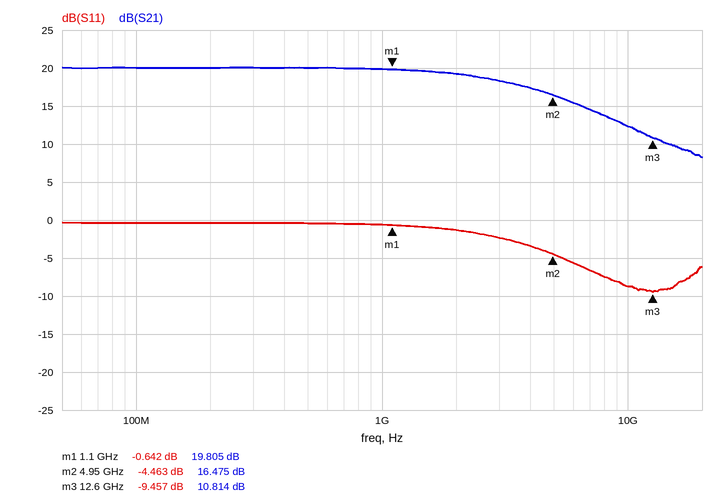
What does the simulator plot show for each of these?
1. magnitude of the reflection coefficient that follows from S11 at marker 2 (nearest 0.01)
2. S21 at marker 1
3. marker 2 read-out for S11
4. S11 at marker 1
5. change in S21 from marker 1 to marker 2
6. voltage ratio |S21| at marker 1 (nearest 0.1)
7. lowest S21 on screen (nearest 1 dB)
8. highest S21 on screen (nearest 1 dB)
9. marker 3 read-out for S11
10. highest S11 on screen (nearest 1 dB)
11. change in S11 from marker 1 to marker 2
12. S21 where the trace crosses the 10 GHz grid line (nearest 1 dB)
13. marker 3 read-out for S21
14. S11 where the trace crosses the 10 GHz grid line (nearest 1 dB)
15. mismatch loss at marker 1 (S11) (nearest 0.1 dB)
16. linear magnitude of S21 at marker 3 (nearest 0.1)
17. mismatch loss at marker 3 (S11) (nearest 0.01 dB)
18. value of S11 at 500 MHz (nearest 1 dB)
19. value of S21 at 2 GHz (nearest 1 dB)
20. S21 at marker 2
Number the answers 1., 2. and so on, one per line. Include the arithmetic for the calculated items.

1. 10^(-4.463/20) ≈ 0.60
2. 19.805 dB
3. -4.463 dB
4. -0.642 dB
5. 16.475 − (19.805) = -3.330 dB
6. 10^(19.805/20) ≈ 9.8
7. 8 dB
8. 20 dB
9. -9.457 dB
10. 0 dB
11. -4.463 − (-0.642) = -3.821 dB
12. 12 dB
13. 10.814 dB
14. -9 dB
15. −10 log10(1 − 10^(-0.642/10)) ≈ 8.6 dB
16. 10^(10.814/20) ≈ 3.5
17. −10 log10(1 − 10^(-9.457/10)) ≈ 0.52 dB
18. 0 dB
19. 19 dB
20. 16.475 dB
